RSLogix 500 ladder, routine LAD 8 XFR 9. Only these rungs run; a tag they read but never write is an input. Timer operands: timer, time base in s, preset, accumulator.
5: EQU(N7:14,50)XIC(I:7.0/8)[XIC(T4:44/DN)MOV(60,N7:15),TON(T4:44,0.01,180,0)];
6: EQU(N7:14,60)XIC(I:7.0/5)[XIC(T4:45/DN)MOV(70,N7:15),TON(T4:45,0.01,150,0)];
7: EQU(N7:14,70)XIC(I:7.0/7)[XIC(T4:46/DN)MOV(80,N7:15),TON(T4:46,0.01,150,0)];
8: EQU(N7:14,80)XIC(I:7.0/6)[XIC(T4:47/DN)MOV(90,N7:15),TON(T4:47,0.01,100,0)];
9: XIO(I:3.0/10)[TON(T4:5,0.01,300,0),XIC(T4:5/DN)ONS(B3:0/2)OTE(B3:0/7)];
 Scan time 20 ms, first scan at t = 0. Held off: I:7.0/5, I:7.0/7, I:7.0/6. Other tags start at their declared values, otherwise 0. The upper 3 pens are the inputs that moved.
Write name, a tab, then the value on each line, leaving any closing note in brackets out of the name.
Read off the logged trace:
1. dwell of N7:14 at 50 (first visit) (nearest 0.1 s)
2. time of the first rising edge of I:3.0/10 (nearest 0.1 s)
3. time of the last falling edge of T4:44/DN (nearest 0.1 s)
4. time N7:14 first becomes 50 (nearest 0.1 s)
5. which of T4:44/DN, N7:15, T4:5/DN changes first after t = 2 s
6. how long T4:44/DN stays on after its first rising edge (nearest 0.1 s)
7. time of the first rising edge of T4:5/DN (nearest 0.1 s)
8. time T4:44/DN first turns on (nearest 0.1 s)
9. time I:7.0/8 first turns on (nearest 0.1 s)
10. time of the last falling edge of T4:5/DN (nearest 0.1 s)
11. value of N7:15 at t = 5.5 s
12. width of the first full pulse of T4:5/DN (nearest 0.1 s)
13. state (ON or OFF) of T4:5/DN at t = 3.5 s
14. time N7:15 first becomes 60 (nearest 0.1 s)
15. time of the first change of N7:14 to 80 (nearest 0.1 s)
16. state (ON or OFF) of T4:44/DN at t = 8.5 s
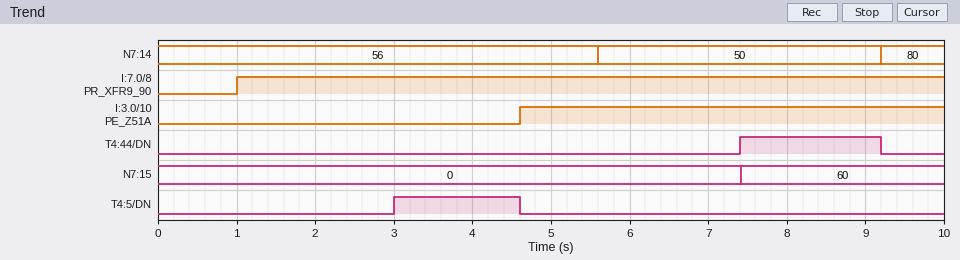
dwell of N7:14 at 50 (first visit)	3.6 s
time of the first rising edge of I:3.0/10	4.6 s
time of the last falling edge of T4:44/DN	9.2 s
time N7:14 first becomes 50	5.6 s
which of T4:44/DN, N7:15, T4:5/DN changes first after t = 2 s	T4:5/DN
how long T4:44/DN stays on after its first rising edge	1.8 s
time of the first rising edge of T4:5/DN	3.0 s
time T4:44/DN first turns on	7.4 s
time I:7.0/8 first turns on	1.0 s
time of the last falling edge of T4:5/DN	4.6 s
value of N7:15 at t = 5.5 s	0
width of the first full pulse of T4:5/DN	1.6 s
state (ON or OFF) of T4:5/DN at t = 3.5 s	ON
time N7:15 first becomes 60	7.4 s
time of the first change of N7:14 to 80	9.2 s
state (ON or OFF) of T4:44/DN at t = 8.5 s	ON
